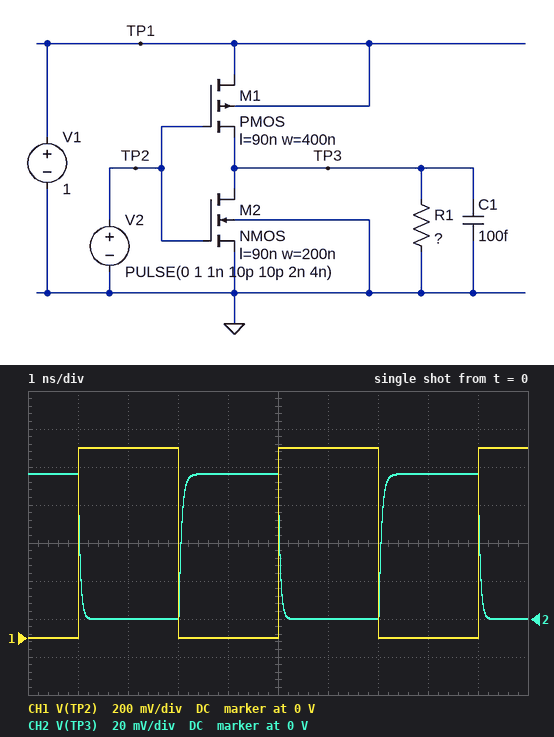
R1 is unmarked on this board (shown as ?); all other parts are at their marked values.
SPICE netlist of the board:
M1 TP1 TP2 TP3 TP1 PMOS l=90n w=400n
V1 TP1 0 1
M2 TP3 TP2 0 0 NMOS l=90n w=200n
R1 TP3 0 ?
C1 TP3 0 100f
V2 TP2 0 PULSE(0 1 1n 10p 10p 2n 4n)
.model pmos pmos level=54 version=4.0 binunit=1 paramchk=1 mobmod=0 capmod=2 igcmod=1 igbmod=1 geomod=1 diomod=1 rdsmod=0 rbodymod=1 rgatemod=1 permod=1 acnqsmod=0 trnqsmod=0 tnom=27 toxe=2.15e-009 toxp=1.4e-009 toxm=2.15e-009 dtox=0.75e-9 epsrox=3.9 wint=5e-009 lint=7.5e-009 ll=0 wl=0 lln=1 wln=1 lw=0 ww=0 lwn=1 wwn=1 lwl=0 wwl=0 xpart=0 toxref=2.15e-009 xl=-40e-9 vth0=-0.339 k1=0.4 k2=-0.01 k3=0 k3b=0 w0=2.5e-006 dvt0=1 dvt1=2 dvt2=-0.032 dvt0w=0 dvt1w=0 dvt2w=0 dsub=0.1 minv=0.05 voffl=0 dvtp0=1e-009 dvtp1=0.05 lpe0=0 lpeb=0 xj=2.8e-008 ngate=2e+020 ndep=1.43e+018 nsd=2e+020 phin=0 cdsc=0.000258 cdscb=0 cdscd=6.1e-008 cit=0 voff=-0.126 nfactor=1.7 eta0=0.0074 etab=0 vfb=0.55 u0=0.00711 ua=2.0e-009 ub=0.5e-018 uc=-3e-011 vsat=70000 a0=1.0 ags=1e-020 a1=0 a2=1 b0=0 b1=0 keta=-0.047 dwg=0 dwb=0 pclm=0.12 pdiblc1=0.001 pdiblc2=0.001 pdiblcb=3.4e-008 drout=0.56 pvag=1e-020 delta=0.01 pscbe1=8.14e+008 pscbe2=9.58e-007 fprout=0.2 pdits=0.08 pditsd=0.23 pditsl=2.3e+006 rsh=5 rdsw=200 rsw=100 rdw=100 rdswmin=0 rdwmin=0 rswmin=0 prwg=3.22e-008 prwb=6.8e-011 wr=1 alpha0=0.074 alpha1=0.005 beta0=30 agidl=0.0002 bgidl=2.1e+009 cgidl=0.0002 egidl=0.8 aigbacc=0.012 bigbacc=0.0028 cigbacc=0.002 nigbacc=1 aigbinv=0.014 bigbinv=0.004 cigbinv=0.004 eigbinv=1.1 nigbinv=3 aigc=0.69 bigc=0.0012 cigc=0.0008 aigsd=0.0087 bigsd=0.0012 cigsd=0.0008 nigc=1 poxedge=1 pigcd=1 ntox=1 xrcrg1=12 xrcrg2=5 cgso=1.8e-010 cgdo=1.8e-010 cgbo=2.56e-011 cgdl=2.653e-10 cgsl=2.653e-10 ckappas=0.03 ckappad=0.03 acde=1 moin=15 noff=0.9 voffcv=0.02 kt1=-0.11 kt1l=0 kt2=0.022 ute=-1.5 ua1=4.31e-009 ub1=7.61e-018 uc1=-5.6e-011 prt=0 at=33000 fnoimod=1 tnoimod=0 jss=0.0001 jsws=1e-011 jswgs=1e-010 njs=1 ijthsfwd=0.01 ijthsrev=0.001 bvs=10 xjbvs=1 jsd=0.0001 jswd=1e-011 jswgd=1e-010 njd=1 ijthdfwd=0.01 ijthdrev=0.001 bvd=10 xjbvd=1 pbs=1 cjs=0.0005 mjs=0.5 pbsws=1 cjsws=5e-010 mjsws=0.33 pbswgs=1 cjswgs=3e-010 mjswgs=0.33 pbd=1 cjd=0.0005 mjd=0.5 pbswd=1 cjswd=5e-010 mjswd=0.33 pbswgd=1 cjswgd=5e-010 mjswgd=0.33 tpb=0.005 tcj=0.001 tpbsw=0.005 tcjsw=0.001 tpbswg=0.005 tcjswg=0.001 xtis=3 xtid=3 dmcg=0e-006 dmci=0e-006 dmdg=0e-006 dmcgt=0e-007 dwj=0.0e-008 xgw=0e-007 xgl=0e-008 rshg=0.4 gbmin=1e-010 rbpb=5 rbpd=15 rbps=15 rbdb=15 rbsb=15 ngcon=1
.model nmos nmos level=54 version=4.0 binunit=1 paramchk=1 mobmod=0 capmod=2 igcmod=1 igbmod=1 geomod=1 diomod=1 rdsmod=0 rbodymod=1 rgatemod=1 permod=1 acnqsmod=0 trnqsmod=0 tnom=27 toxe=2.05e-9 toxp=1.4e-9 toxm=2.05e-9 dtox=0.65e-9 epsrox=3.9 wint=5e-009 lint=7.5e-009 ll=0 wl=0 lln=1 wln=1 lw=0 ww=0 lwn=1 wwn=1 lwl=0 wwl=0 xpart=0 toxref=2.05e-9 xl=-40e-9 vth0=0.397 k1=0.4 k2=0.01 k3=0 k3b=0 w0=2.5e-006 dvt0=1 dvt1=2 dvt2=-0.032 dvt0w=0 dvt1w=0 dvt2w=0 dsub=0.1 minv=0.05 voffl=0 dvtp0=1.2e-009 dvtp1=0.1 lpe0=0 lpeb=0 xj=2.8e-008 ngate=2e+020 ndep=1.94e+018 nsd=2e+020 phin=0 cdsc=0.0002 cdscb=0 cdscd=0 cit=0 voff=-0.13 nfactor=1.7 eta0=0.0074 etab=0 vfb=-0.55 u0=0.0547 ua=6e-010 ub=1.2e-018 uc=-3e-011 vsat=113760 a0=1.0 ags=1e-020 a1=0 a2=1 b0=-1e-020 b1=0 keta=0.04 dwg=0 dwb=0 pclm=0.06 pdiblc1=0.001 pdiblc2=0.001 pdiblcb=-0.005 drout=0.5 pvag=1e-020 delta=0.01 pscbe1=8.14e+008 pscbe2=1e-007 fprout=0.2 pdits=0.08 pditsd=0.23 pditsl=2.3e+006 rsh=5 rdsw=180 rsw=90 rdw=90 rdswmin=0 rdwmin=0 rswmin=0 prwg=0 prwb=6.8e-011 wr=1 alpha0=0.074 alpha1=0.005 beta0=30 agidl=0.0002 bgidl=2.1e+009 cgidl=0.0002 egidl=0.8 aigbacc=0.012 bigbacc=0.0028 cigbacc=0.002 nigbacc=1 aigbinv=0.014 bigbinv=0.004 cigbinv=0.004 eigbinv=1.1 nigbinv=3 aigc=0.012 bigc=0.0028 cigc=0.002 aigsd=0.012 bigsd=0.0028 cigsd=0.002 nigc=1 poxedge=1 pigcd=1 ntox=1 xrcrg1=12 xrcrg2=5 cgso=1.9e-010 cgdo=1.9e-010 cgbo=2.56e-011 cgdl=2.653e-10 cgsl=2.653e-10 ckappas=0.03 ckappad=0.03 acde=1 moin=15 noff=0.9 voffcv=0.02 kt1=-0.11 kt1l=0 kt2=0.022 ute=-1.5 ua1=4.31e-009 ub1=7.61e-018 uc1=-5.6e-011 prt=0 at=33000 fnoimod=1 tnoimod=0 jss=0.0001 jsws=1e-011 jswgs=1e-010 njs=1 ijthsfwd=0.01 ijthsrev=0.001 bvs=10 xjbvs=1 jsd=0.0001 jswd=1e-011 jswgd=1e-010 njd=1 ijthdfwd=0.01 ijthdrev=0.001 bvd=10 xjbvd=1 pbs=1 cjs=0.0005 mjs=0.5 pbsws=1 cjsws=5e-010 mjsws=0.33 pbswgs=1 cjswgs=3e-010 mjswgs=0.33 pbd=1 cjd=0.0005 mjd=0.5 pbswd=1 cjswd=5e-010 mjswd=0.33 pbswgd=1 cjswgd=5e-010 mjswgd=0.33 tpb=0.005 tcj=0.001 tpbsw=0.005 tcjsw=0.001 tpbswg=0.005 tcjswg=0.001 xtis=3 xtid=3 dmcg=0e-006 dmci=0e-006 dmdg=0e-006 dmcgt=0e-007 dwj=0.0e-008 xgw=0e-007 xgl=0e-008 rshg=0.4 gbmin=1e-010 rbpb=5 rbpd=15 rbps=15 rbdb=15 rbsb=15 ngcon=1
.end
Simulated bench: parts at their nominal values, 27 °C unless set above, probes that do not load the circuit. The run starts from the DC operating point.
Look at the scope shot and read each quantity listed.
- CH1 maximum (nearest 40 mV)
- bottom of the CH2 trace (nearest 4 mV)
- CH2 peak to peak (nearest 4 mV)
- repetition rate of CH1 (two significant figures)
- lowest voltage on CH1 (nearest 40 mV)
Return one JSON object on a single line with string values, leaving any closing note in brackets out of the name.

{"CH1 maximum": "1.00 V", "bottom of the CH2 trace": "0 V", "CH2 peak to peak": "76 mV", "repetition rate of CH1": "250 MHz", "lowest voltage on CH1": "0 V"}
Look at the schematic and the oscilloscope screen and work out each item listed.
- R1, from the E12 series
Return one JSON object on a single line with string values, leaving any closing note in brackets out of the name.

{"R1, from the E12 series": "560 Ω"}
